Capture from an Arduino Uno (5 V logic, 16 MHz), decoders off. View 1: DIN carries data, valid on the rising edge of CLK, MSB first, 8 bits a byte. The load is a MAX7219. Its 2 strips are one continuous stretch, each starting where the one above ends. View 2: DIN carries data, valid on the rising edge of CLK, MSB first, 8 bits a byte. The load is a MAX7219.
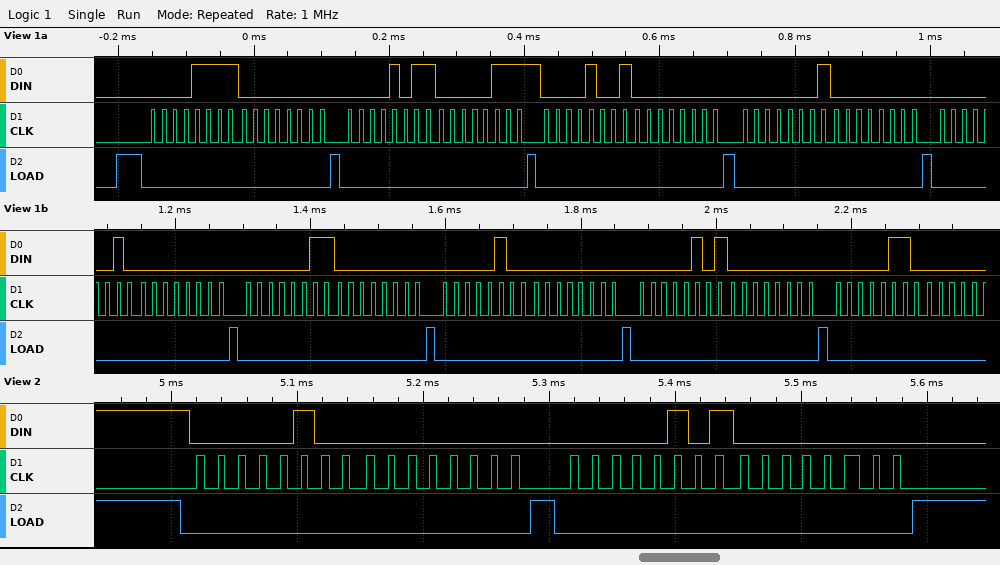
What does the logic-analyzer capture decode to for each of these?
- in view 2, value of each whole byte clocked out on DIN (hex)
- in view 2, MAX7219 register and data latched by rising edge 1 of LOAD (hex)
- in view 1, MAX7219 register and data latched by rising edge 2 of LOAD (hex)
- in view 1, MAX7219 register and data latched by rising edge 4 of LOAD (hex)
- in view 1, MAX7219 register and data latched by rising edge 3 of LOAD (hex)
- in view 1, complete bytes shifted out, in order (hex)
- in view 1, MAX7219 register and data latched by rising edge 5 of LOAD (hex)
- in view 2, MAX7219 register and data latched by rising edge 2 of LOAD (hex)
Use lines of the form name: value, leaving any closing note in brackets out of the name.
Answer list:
in view 2, value of each whole byte clocked out on DIN: 04 00 05 00
in view 2, MAX7219 register and data latched by rising edge 1 of LOAD: register 0x4, data 0x00
in view 1, MAX7219 register and data latched by rising edge 2 of LOAD: register 0xF, data 0x00
in view 1, MAX7219 register and data latched by rising edge 4 of LOAD: register 0x9, data 0x00
in view 1, MAX7219 register and data latched by rising edge 3 of LOAD: register 0xB, data 0x07
in view 1, complete bytes shifted out, in order: 0F 00 0B 07 09 00 01 00 02 00 03 00 04 00 05 00 06
in view 1, MAX7219 register and data latched by rising edge 5 of LOAD: register 0x1, data 0x00
in view 2, MAX7219 register and data latched by rising edge 2 of LOAD: register 0x5, data 0x00
